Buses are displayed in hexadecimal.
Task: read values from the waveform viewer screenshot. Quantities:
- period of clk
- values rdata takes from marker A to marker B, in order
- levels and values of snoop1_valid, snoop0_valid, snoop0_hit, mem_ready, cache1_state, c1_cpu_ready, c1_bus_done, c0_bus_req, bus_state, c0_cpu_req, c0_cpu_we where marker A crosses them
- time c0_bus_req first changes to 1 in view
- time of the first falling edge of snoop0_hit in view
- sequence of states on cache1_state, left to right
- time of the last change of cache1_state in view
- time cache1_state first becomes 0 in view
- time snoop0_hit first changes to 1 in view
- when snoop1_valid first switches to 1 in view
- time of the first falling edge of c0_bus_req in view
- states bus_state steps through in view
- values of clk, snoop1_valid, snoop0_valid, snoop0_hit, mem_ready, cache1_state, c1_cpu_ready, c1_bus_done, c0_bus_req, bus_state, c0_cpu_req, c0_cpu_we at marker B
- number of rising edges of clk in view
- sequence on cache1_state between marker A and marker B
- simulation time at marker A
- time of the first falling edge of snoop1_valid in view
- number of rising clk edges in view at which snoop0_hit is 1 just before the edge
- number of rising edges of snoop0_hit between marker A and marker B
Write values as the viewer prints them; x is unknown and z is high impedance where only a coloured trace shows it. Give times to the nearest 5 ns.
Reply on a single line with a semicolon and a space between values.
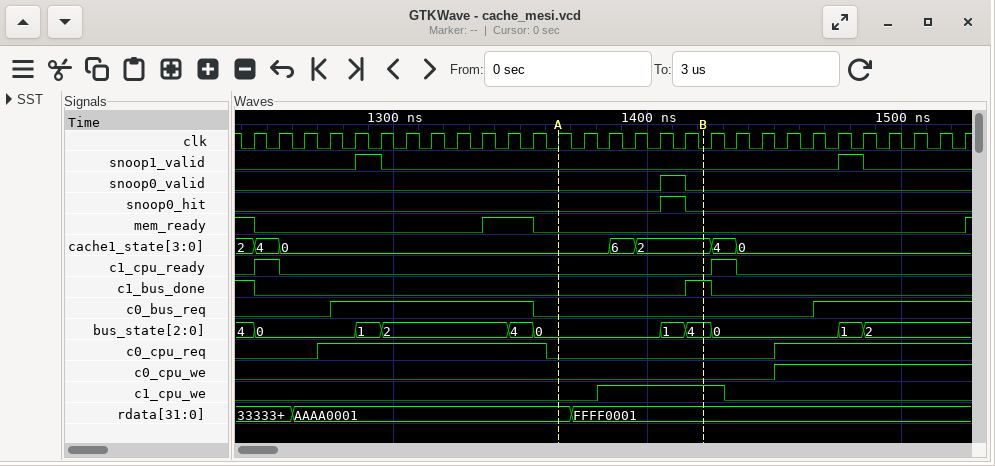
10 ns; AAAA0001, FFFF0001; snoop1_valid=0, snoop0_valid=0, snoop0_hit=0, mem_ready=0, cache1_state=0, c1_cpu_ready=0, c1_bus_done=0, c0_bus_req=0, bus_state=0, c0_cpu_req=0, c0_cpu_we=0; 1275 ns; 1415 ns; 2, 4, 0, 6, 2, 4, 0; 1435 ns; 1255 ns; 1405 ns; 1285 ns; 1355 ns; 4, 0, 1, 2, 4, 0, 1, 4, 0, 1, 2; clk=0, snoop1_valid=0, snoop0_valid=0, snoop0_hit=0, mem_ready=0, cache1_state=2, c1_cpu_ready=0, c1_bus_done=1, c0_bus_req=0, bus_state=4, c0_cpu_req=0, c0_cpu_we=0; 29; 0, 6, 2; 1365 ns; 1295 ns; 1; 1
